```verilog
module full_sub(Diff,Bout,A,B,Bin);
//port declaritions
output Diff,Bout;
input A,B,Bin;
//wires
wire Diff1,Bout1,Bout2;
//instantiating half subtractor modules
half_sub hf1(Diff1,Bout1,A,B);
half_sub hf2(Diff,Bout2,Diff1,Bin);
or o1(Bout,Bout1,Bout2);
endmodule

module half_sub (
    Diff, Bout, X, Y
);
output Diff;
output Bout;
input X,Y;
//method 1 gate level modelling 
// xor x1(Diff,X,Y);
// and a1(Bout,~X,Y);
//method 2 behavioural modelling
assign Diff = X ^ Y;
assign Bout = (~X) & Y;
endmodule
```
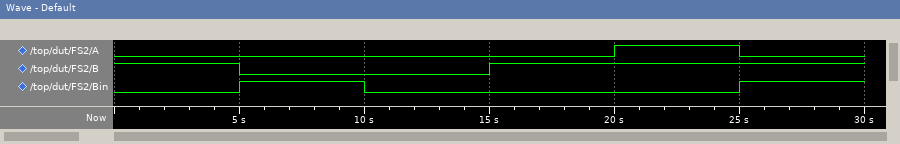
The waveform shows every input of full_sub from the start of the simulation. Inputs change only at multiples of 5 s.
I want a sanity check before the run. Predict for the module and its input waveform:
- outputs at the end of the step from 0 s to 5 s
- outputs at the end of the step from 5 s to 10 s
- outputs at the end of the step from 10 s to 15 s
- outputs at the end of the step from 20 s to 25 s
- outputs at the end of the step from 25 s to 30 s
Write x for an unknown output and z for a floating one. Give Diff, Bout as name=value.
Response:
Diff=1, Bout=1
Diff=1, Bout=1
Diff=0, Bout=0
Diff=0, Bout=0
Diff=0, Bout=1
